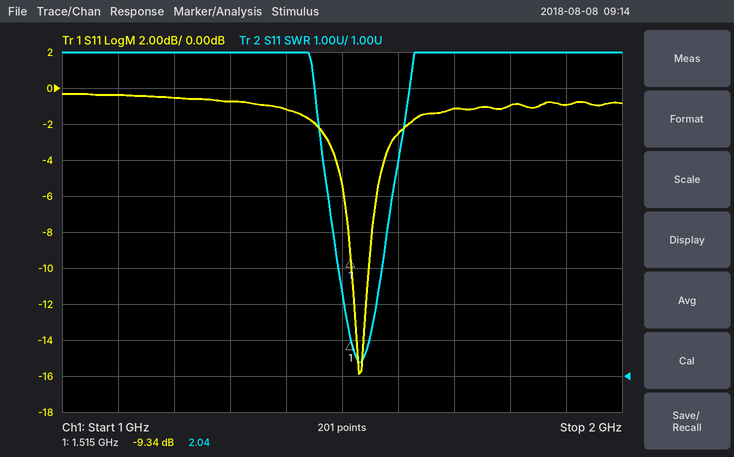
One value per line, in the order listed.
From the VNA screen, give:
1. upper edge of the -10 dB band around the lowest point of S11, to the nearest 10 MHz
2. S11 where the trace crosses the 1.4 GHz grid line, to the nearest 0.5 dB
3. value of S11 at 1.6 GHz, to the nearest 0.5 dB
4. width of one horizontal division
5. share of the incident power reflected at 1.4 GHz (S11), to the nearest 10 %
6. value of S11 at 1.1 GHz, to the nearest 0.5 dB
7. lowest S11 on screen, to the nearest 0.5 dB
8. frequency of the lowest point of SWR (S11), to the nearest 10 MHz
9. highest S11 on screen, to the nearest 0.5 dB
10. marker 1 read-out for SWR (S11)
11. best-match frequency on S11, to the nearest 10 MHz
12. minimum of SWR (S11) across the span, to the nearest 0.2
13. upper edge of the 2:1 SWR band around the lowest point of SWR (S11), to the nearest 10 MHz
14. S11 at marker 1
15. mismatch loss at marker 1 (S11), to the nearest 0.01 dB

1.55 GHz
-1.0 dB
-2.5 dB
100 MHz
80 %
-0.5 dB
-16.0 dB
1.53 GHz
-0.5 dB
2.04
1.53 GHz
1.4
1.55 GHz
-9.34 dB
0.54 dB
